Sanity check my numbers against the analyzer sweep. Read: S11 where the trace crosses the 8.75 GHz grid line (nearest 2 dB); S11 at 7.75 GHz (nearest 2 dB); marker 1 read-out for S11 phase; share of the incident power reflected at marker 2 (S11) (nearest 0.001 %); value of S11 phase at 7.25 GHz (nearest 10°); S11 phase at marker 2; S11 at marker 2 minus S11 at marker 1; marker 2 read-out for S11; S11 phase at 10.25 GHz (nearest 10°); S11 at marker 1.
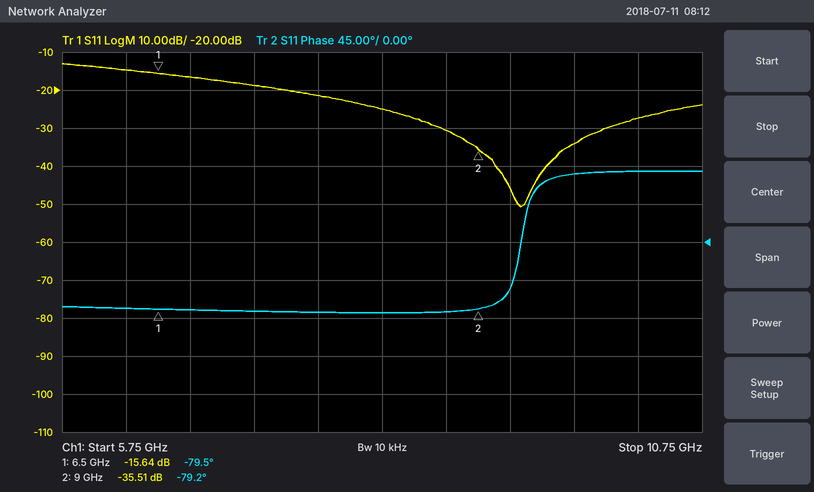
-30 dB
-22 dB
-79.5°
0.028 %
-80°
-79.2°
-19.87 dB
-35.51 dB
80°
-15.64 dB
